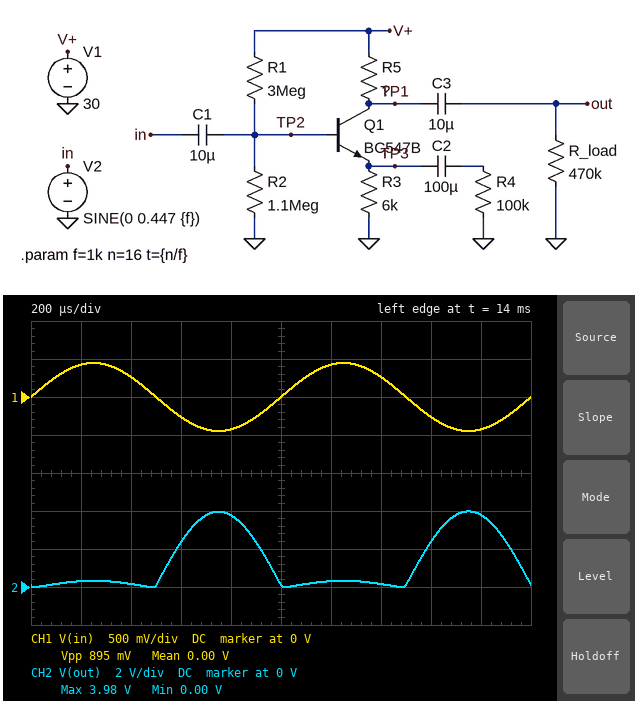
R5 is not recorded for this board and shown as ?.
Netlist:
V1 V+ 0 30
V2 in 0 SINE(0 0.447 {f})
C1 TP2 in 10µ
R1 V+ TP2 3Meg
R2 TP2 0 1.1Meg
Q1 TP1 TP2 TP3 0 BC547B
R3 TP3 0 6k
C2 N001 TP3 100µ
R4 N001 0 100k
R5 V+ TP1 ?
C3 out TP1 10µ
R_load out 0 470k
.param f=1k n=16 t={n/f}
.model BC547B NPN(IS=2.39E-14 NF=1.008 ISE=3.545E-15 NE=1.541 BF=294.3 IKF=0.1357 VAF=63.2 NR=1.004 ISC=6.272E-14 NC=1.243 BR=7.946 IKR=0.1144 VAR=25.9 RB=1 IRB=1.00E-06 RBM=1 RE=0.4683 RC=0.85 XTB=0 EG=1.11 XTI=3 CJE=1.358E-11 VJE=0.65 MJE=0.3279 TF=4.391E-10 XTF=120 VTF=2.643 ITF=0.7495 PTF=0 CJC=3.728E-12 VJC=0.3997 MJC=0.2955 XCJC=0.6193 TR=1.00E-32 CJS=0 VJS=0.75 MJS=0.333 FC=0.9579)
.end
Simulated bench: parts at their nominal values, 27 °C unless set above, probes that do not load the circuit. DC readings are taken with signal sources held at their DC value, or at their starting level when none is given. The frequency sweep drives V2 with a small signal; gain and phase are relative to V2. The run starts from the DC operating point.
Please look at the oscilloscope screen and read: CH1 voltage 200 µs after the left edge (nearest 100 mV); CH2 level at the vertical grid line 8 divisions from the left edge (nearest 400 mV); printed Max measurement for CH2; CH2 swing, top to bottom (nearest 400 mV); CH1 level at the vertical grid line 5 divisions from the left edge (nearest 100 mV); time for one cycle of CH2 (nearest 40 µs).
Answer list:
400 mV
2.4 V
3.98 V
4.0 V
0 V
1.00 ms
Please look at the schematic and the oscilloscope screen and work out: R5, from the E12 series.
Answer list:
56 kΩ
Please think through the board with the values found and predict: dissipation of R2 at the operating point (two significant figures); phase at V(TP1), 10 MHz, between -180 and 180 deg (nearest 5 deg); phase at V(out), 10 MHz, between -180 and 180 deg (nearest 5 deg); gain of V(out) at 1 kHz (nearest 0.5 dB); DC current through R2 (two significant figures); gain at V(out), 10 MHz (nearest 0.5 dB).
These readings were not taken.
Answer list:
11 µW
5 deg
5 deg
-16.0 dB
3.2 µA
0 dB
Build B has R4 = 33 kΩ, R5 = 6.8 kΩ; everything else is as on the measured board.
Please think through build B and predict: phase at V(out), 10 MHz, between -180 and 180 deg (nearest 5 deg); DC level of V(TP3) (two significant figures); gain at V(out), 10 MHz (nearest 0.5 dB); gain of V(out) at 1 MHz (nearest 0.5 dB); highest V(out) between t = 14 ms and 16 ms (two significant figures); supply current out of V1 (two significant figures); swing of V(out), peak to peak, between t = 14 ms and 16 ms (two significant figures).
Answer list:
125 deg
5.4 V
2.0 dB
2.5 dB
580 mV
910 µA
1.2 V
